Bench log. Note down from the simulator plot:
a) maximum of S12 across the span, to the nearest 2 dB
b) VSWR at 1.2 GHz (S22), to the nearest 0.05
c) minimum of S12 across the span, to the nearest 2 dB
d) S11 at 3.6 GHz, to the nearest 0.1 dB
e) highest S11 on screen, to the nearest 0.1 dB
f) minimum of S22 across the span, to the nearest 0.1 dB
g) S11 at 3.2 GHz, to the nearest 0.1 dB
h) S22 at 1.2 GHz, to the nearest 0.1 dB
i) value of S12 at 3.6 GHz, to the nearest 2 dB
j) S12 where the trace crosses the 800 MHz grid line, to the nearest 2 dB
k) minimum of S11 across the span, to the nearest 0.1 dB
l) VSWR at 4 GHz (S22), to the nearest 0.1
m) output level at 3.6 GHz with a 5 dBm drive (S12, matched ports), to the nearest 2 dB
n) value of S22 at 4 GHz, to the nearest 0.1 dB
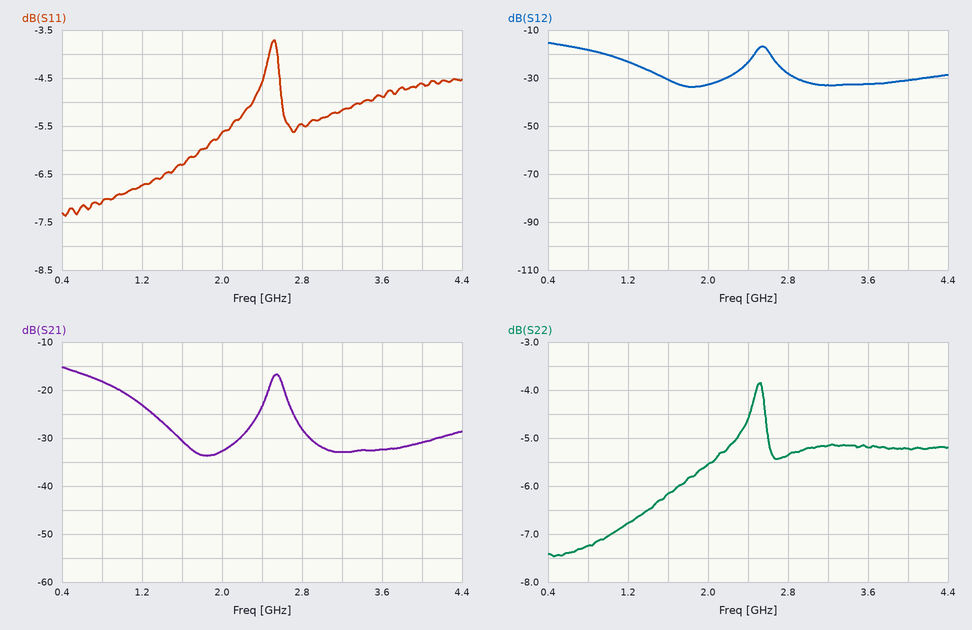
-16 dB
2.70
-34 dB
-4.9 dB
-3.7 dB
-7.5 dB
-5.2 dB
-6.8 dB
-32 dB
-18 dB
-7.4 dB
3.4
-28 dBm
-5.2 dB
